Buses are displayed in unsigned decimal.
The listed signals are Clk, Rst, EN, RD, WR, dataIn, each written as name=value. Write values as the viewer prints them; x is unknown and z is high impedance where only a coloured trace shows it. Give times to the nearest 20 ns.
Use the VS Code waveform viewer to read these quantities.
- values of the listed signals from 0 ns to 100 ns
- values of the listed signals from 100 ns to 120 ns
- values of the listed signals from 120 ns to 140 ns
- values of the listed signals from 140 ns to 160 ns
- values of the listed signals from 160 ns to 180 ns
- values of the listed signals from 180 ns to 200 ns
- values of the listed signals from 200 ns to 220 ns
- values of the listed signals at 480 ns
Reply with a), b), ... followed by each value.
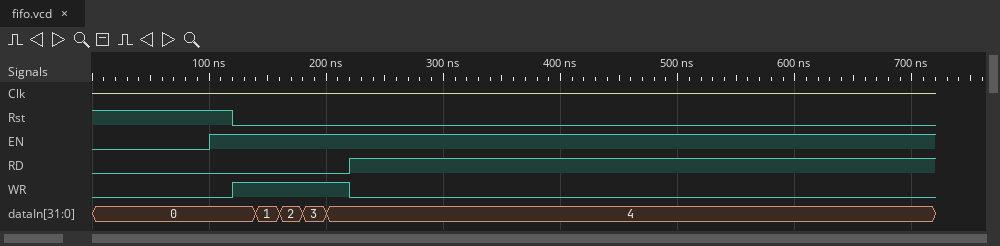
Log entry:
a) Clk=z, Rst=1, EN=0, RD=0, WR=0, dataIn=0
b) Clk=z, Rst=1, EN=1, RD=0, WR=0, dataIn=0
c) Clk=z, Rst=0, EN=1, RD=0, WR=1, dataIn=0
d) Clk=z, Rst=0, EN=1, RD=0, WR=1, dataIn=1
e) Clk=z, Rst=0, EN=1, RD=0, WR=1, dataIn=2
f) Clk=z, Rst=0, EN=1, RD=0, WR=1, dataIn=3
g) Clk=z, Rst=0, EN=1, RD=0, WR=1, dataIn=4
h) Clk=z, Rst=0, EN=1, RD=1, WR=0, dataIn=4
